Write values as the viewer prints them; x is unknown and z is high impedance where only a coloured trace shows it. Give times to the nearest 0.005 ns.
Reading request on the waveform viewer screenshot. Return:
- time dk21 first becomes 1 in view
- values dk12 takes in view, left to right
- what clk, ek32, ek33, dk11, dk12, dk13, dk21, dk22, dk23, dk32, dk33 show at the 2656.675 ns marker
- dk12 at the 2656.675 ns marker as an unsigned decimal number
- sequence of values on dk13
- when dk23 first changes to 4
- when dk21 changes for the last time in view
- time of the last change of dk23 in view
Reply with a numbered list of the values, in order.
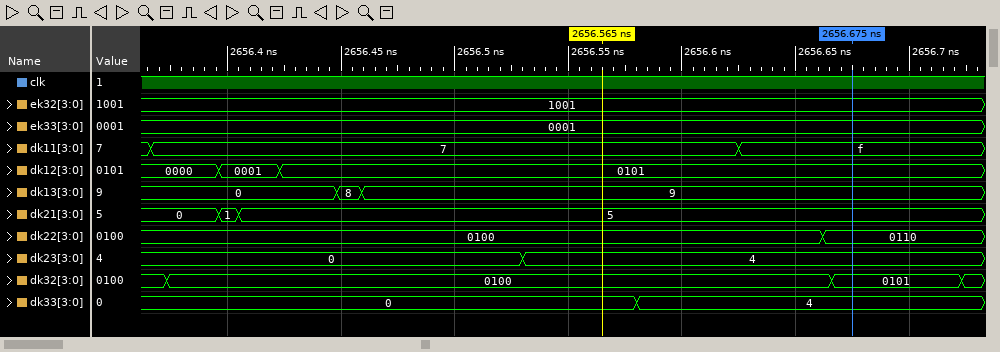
1. 2656.395 ns
2. 0000, 0001, 0101
3. clk=1, ek32=1001, ek33=0001, dk11=f, dk12=0101, dk13=9, dk21=5, dk22=0110, dk23=4, dk32=0101, dk33=4
4. 5
5. 0, 8, 9
6. 2656.53 ns
7. 2656.405 ns
8. 2656.53 ns
